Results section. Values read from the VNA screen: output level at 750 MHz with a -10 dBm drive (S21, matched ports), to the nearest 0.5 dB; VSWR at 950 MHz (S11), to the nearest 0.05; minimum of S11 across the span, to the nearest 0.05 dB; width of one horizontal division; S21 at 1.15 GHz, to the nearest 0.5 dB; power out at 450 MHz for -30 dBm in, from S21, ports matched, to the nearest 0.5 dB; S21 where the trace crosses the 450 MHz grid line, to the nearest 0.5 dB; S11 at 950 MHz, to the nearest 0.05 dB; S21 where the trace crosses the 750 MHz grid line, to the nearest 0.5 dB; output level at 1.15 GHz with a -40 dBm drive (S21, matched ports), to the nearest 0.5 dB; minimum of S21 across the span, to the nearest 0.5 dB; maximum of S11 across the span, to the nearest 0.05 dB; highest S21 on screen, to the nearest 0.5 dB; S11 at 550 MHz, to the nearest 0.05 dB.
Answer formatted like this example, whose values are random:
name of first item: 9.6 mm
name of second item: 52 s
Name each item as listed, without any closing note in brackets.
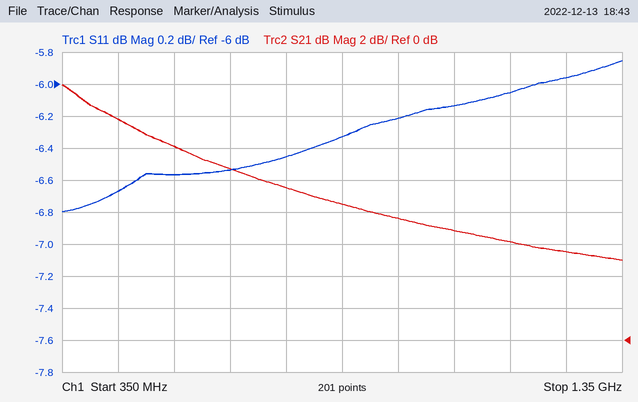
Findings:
output level at 750 MHz with a -10 dBm drive (S21, matched ports), to the nearest 0.5 dB: -0.5 dBm
VSWR at 950 MHz (S11), to the nearest 0.05: 2.90
minimum of S11 across the span, to the nearest 0.05 dB: -6.80 dB
width of one horizontal division: 100 MHz
S21 at 1.15 GHz, to the nearest 0.5 dB: 6.0 dB
power out at 450 MHz for -30 dBm in, from S21, ports matched, to the nearest 0.5 dB: -16.0 dBm
S21 where the trace crosses the 450 MHz grid line, to the nearest 0.5 dB: 14.0 dB
S11 at 950 MHz, to the nearest 0.05 dB: -6.20 dB
S21 where the trace crosses the 750 MHz grid line, to the nearest 0.5 dB: 9.5 dB
output level at 1.15 GHz with a -40 dBm drive (S21, matched ports), to the nearest 0.5 dB: -34.0 dBm
minimum of S21 across the span, to the nearest 0.5 dB: 5.0 dB
maximum of S11 across the span, to the nearest 0.05 dB: -5.85 dB
highest S21 on screen, to the nearest 0.5 dB: 16.0 dB
S11 at 550 MHz, to the nearest 0.05 dB: -6.55 dB
